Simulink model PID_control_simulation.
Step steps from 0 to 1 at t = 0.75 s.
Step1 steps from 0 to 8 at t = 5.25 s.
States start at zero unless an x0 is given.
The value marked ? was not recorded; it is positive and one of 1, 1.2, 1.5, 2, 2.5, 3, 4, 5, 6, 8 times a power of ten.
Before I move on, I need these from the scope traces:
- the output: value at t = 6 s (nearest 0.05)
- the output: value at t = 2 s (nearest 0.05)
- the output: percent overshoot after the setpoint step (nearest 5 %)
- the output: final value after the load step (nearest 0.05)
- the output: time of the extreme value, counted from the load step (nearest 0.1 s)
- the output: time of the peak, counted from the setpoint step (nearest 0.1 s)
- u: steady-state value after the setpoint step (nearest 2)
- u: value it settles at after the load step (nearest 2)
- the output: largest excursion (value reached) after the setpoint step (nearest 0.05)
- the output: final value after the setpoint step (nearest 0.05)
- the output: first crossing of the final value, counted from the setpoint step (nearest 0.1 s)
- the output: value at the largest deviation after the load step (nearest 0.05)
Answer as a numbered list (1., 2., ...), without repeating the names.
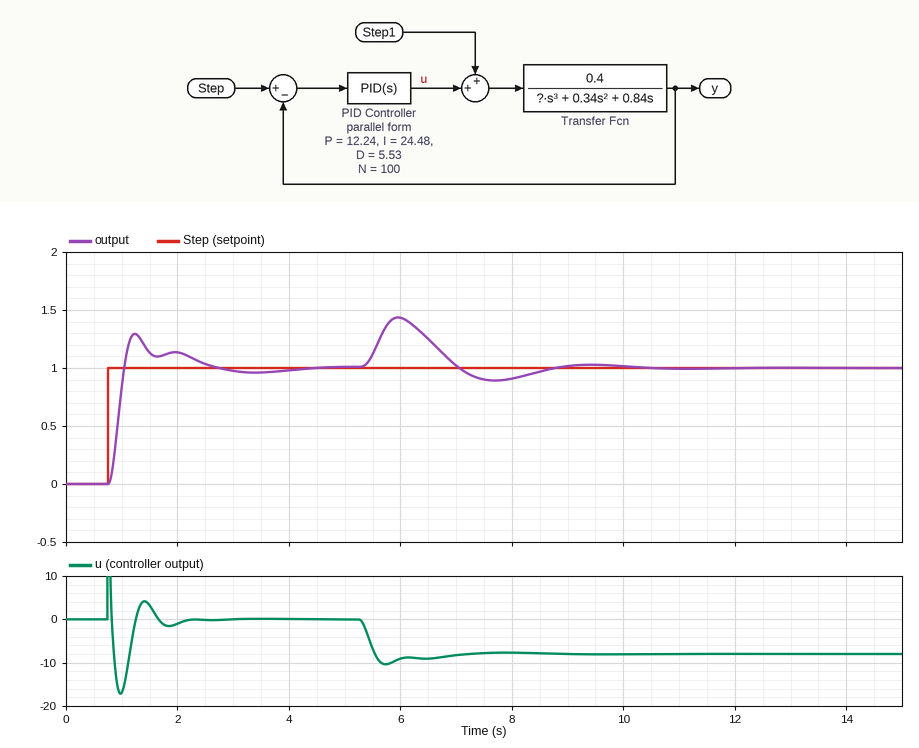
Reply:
1. 1.45
2. 1.15
3. 30 %
4. 1.00
5. 0.7 s
6. 0.5 s
7. 0
8. -8
9. 1.30
10. 1.00
11. 0.3 s
12. 1.45
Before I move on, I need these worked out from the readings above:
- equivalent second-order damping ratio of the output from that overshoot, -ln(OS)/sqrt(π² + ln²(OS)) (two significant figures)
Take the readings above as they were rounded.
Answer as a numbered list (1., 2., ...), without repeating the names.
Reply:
1. 0.36
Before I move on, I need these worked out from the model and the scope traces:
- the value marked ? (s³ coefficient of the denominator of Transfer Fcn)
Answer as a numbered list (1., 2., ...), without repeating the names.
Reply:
1. 0.04
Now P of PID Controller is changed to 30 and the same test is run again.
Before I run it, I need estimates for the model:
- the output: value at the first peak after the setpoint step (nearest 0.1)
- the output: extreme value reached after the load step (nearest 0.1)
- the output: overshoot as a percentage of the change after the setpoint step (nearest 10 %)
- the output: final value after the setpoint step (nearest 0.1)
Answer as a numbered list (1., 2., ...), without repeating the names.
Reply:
1. 1.6
2. 1.3
3. 60 %
4. 1.0
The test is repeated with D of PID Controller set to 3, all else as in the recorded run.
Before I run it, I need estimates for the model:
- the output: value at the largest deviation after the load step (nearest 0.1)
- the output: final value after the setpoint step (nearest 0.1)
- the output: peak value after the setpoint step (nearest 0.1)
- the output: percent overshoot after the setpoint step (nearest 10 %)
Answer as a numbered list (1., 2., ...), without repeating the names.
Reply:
1. 1.6
2. 1.0
3. 1.5
4. 50 %
